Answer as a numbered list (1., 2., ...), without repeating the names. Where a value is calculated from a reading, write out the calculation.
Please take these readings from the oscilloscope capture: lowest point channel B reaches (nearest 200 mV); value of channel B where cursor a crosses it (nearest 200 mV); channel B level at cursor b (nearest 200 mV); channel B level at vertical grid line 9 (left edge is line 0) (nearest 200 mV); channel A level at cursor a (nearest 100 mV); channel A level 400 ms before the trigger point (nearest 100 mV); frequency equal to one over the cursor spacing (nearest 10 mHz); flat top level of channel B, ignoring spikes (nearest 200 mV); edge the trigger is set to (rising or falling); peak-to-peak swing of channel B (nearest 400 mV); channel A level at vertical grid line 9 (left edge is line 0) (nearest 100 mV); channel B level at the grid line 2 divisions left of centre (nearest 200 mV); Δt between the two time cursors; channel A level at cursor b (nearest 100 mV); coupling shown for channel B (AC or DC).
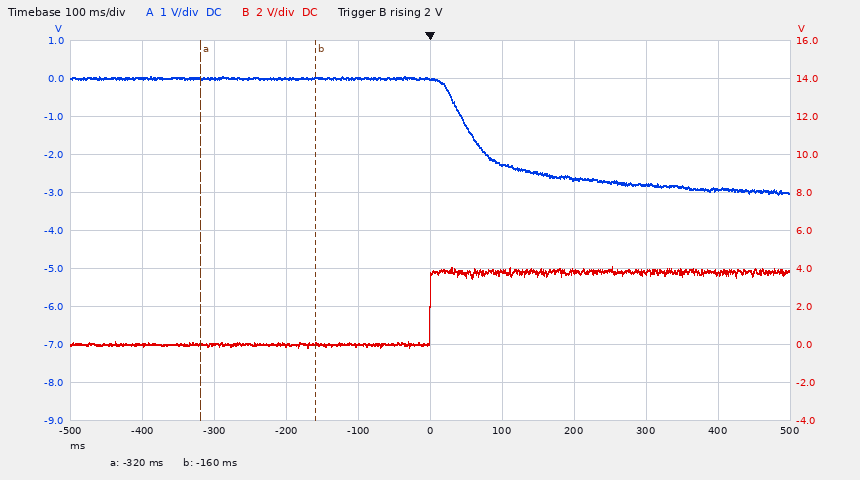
1. -200 mV
2. 0.0 V
3. 0.0 V
4. 3.8 V
5. 0.0 V
6. 0.0 V
7. 1 / 160 ms ≈ 6.25 Hz
8. 3.8 V
9. rising
10. 4.4 V
11. -2.9 V
12. 0.0 V
13. -160 ms − (-320 ms) = 160 ms
14. 0.0 V
15. DC
